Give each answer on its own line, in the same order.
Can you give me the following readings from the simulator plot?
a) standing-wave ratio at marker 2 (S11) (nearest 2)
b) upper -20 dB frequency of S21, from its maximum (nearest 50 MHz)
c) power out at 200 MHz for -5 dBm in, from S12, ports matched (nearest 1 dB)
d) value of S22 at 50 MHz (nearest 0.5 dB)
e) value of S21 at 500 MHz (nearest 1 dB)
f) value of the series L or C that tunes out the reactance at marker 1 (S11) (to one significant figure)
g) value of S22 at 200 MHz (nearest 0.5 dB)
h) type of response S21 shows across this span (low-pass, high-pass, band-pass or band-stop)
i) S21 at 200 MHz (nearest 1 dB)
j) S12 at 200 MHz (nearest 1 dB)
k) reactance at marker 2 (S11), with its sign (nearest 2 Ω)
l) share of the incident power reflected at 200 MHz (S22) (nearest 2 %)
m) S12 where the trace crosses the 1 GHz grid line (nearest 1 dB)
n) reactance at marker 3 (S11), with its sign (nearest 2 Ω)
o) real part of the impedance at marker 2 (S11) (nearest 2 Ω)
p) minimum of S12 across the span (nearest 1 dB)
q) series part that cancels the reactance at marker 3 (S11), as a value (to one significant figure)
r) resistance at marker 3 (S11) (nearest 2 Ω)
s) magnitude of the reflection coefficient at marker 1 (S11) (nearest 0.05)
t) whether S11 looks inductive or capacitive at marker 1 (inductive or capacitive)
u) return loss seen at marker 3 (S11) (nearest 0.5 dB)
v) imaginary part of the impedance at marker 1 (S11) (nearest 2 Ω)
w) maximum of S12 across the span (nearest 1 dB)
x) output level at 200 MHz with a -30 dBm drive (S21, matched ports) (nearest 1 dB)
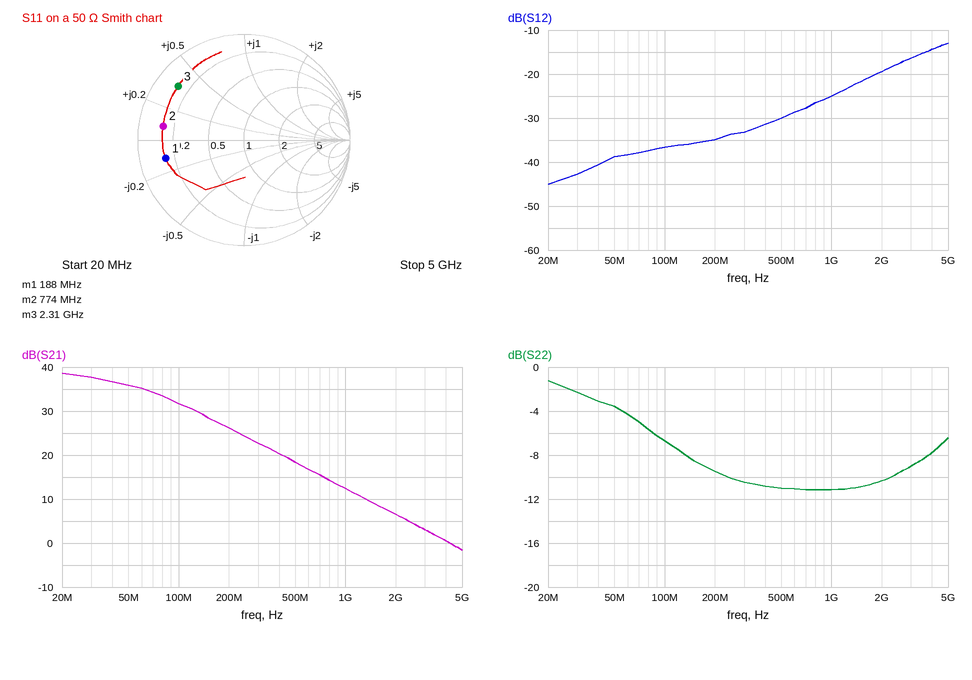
8
500 MHz
-40 dBm
-3.5 dB
18 dB
5 nH
-9.5 dB
low-pass
26 dB
-35 dB
+4 Ω
12 %
-25 dB
+18 Ω
6 Ω
-45 dB
4 pF
6 Ω
0.75
capacitive
2.0 dB
-6 Ω
-13 dB
-4 dBm
